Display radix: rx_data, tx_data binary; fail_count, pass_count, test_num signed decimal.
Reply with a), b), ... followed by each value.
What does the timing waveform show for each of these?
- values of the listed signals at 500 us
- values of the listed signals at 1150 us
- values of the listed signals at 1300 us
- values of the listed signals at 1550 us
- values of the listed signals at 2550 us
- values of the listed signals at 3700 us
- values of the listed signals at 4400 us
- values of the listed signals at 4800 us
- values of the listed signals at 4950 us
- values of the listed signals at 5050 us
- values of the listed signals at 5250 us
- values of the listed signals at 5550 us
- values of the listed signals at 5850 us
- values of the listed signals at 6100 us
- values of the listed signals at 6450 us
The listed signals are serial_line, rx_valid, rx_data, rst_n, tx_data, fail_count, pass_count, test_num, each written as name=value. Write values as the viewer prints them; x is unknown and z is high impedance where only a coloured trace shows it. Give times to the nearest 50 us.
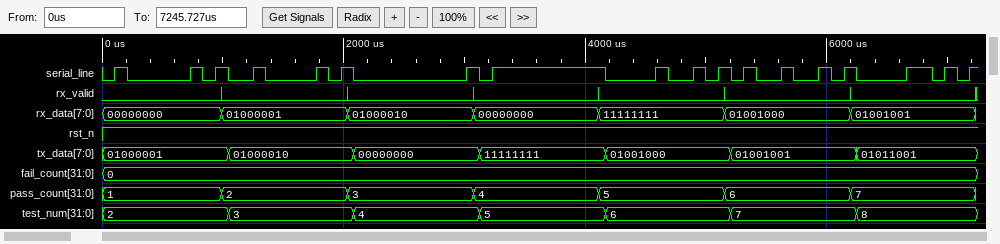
a) serial_line=0, rx_valid=0, rx_data=00000000, rst_n=1, tx_data=01000001, fail_count=0, pass_count=1, test_num=2
b) serial_line=0, rx_valid=0, rx_data=01000001, rst_n=1, tx_data=01000010, fail_count=0, pass_count=2, test_num=3
c) serial_line=1, rx_valid=0, rx_data=01000001, rst_n=1, tx_data=01000010, fail_count=0, pass_count=2, test_num=3
d) serial_line=0, rx_valid=0, rx_data=01000001, rst_n=1, tx_data=01000010, fail_count=0, pass_count=2, test_num=3
e) serial_line=0, rx_valid=0, rx_data=01000010, rst_n=1, tx_data=00000000, fail_count=0, pass_count=3, test_num=4
f) serial_line=1, rx_valid=0, rx_data=00000000, rst_n=1, tx_data=11111111, fail_count=0, pass_count=4, test_num=5
g) serial_line=0, rx_valid=0, rx_data=11111111, rst_n=1, tx_data=01001000, fail_count=0, pass_count=5, test_num=6
h) serial_line=0, rx_valid=0, rx_data=11111111, rst_n=1, tx_data=01001000, fail_count=0, pass_count=5, test_num=6
i) serial_line=1, rx_valid=0, rx_data=11111111, rst_n=1, tx_data=01001000, fail_count=0, pass_count=5, test_num=6
j) serial_line=0, rx_valid=0, rx_data=11111111, rst_n=1, tx_data=01001000, fail_count=0, pass_count=5, test_num=6
k) serial_line=0, rx_valid=0, rx_data=01001000, rst_n=1, tx_data=01001001, fail_count=0, pass_count=6, test_num=7
l) serial_line=0, rx_valid=0, rx_data=01001000, rst_n=1, tx_data=01001001, fail_count=0, pass_count=6, test_num=7
m) serial_line=0, rx_valid=0, rx_data=01001000, rst_n=1, tx_data=01001001, fail_count=0, pass_count=6, test_num=7
n) serial_line=0, rx_valid=0, rx_data=01001000, rst_n=1, tx_data=01001001, fail_count=0, pass_count=6, test_num=7
o) serial_line=0, rx_valid=0, rx_data=01001001, rst_n=1, tx_data=01011001, fail_count=0, pass_count=7, test_num=8
